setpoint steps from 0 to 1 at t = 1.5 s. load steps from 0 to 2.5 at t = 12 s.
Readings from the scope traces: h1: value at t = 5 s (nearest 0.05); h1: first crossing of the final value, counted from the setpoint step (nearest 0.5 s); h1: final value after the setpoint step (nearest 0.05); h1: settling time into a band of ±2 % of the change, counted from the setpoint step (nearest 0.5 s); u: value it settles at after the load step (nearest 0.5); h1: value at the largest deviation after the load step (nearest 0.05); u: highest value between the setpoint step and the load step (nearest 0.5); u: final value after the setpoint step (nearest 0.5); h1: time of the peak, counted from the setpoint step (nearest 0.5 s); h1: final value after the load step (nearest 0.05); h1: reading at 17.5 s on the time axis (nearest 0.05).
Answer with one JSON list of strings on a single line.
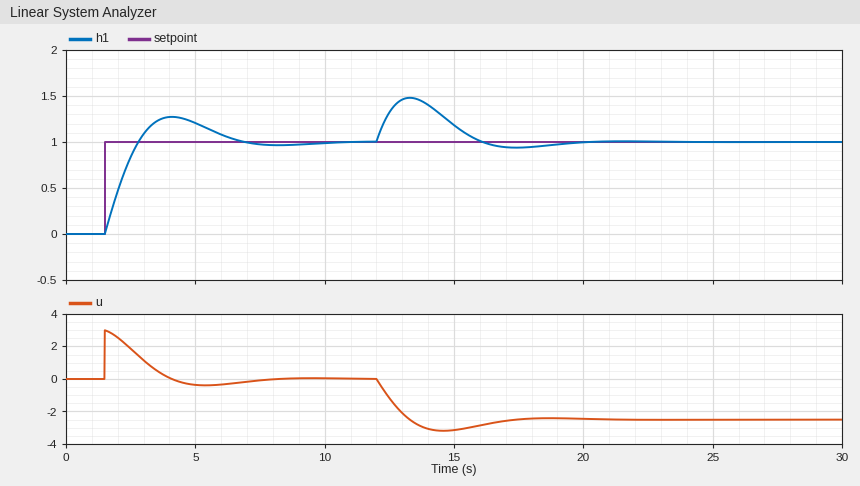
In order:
["1.20", "1.5 s", "1.00", "8.0 s", "-2.5", "1.50", "3.0", "0.0", "2.5 s", "1.00", "0.95"]
